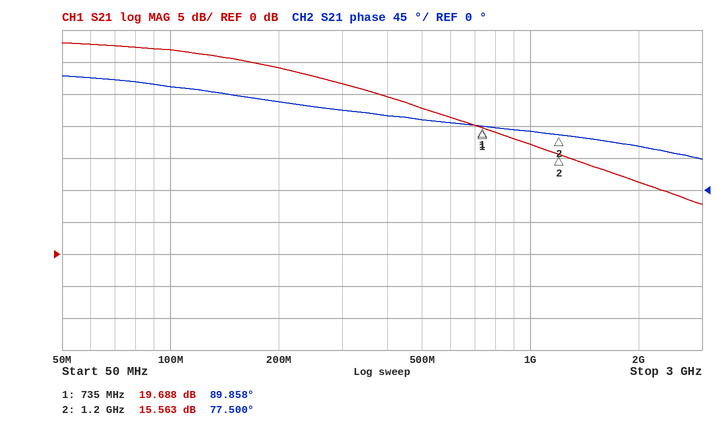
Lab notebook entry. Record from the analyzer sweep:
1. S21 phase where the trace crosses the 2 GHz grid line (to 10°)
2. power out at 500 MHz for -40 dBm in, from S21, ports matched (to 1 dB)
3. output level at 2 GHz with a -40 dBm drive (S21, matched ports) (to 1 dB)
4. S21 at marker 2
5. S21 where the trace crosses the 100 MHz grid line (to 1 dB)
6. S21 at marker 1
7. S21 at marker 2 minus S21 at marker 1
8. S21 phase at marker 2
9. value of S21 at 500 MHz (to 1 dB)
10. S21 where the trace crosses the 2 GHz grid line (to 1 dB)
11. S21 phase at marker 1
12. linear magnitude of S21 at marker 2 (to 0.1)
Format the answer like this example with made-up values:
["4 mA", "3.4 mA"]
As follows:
["60°", "-17 dBm", "-29 dBm", "15.563 dB", "32 dB", "19.688 dB", "-4.125 dB", "77.500°", "23 dB", "11 dB", "89.858°", "6.0"]
